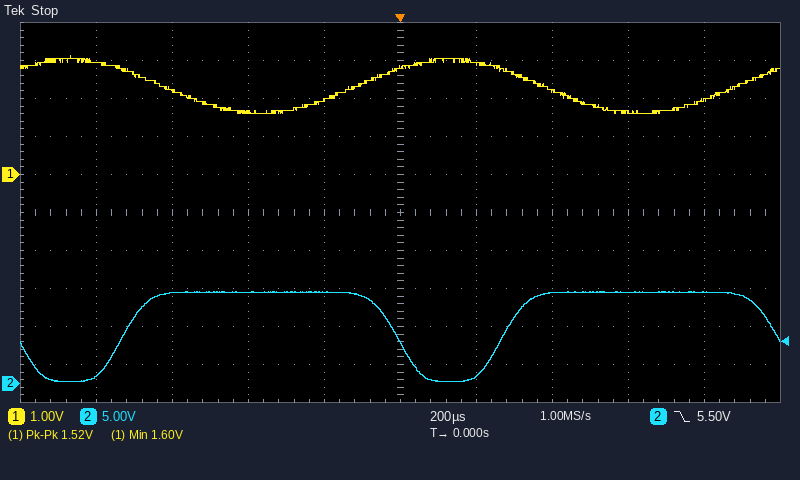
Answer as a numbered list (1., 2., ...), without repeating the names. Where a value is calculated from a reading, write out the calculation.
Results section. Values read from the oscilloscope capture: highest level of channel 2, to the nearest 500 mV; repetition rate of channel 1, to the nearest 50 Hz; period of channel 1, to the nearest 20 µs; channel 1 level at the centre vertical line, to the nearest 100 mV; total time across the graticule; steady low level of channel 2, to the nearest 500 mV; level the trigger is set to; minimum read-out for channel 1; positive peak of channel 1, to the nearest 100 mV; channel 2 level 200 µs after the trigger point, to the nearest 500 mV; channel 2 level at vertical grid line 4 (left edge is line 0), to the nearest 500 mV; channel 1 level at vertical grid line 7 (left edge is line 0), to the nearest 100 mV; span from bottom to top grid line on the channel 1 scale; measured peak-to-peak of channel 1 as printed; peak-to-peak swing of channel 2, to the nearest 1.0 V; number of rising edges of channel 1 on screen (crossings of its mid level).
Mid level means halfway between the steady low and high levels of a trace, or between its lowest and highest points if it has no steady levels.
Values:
1. 12.0 V
2. 1 / 1.00 ms ≈ 1.00 kHz
3. 1.00 ms
4. 2.8 V
5. 2 ms
6. 500 mV
7. 5.50 V
8. 1.60 V
9. 3.1 V
10. 1.0 V
11. 12.0 V
12. 2.2 V
13. 10 V
14. 1.52 V
15. 12.0 V
16. 2
